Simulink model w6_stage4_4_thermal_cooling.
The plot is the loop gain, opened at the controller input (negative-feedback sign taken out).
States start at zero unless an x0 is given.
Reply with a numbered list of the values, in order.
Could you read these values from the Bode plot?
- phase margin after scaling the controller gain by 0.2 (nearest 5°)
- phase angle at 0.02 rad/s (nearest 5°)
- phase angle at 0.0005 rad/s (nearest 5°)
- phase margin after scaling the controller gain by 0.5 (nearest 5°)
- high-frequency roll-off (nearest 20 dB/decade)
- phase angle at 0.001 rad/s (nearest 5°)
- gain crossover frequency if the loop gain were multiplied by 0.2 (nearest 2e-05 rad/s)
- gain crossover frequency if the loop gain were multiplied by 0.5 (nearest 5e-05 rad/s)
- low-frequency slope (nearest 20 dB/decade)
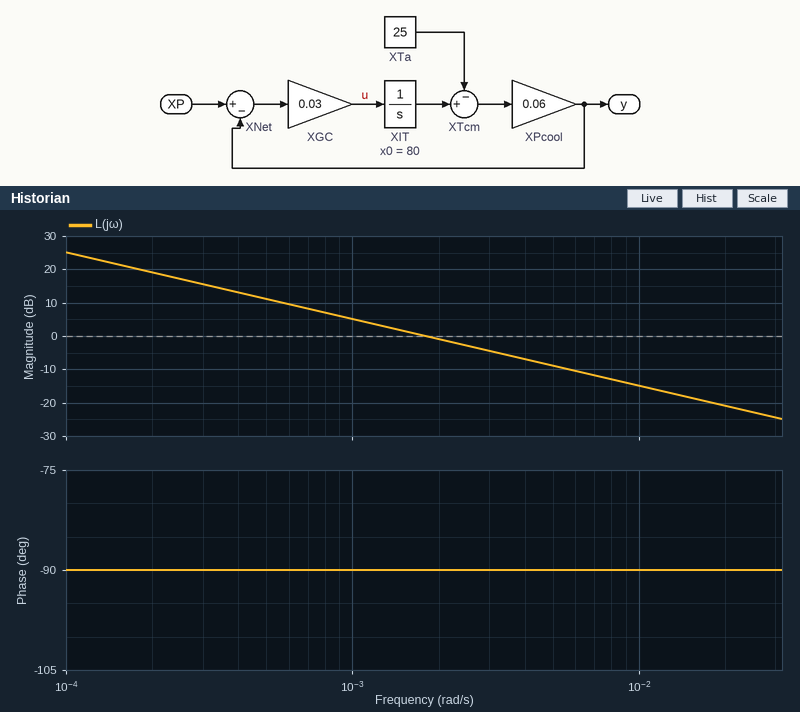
1. 90°
2. -90°
3. -90°
4. 90°
5. -20 dB/decade
6. -90°
7. 0.00036 rad/s
8. 0.00090 rad/s
9. -20 dB/decade
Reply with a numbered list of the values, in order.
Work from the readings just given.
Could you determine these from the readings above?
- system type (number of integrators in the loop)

1. 1
